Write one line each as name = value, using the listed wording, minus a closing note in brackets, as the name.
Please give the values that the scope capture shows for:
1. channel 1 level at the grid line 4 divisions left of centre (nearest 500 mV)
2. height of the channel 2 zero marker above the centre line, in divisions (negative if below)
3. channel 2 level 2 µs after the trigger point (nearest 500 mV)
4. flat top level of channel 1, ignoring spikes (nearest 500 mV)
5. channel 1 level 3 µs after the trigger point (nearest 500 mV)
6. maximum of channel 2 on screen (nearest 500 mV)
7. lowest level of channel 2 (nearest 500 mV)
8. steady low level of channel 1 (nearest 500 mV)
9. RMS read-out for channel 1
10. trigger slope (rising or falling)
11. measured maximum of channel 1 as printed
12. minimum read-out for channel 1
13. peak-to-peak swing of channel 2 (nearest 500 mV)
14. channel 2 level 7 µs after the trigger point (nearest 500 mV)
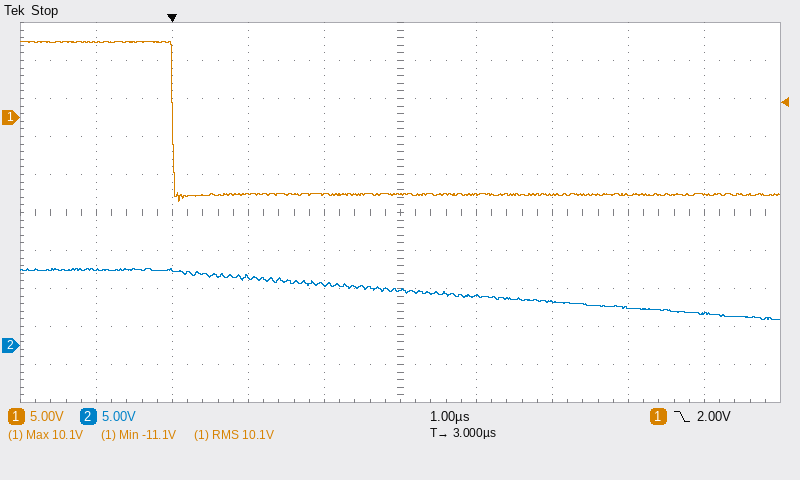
channel 1 level at the grid line 4 divisions left of centre = 10.0 V
height of the channel 2 zero marker above the centre line, in divisions = -3.5 div
channel 2 level 2 µs after the trigger point = 8.0 V
flat top level of channel 1, ignoring spikes = 10.0 V
channel 1 level 3 µs after the trigger point = -10.0 V
maximum of channel 2 on screen = 10.0 V
lowest level of channel 2 = 3.5 V
steady low level of channel 1 = -10.0 V
RMS read-out for channel 1 = 10.1 V
trigger slope = falling
measured maximum of channel 1 as printed = 10.1 V
minimum read-out for channel 1 = -11.1 V
peak-to-peak swing of channel 2 = 6.5 V
channel 2 level 7 µs after the trigger point = 4.0 V
